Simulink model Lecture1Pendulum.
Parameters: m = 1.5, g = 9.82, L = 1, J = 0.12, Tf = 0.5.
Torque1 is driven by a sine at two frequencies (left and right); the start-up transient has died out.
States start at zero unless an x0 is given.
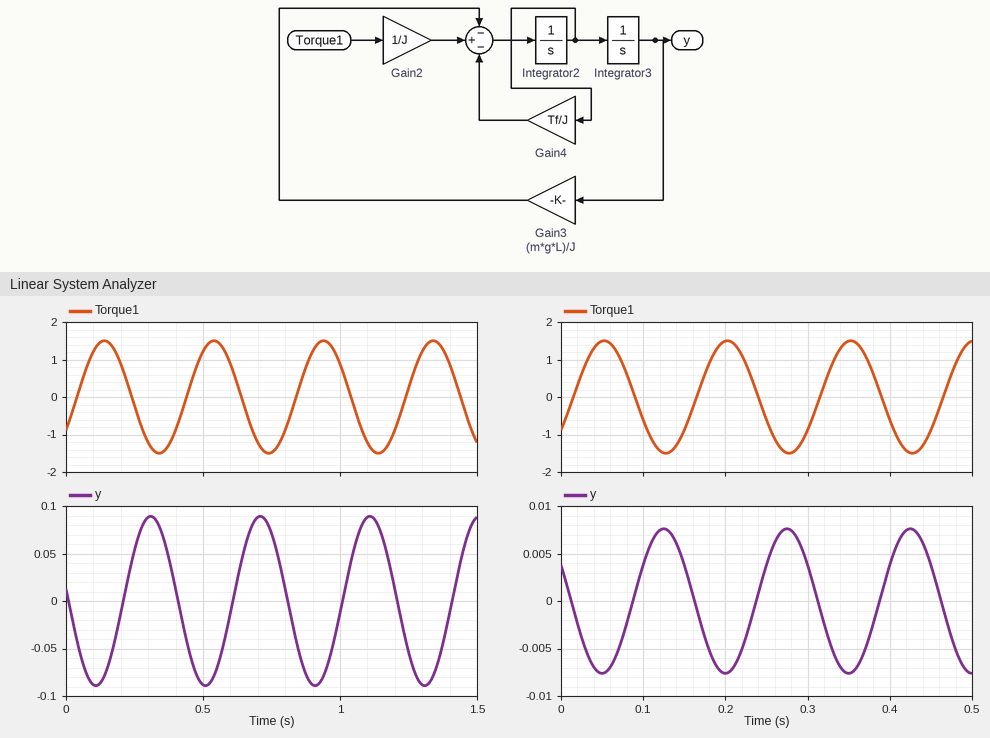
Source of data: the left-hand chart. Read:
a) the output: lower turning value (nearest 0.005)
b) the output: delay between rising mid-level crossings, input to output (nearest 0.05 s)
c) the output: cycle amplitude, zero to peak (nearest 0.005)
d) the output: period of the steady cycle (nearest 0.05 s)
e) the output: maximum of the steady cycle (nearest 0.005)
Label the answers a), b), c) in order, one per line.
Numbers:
a) -0.090
b) 0.15 s
c) 0.090
d) 0.40 s
e) 0.090
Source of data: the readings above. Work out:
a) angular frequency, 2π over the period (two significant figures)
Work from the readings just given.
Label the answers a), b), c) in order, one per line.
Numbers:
a) 16 rad/s
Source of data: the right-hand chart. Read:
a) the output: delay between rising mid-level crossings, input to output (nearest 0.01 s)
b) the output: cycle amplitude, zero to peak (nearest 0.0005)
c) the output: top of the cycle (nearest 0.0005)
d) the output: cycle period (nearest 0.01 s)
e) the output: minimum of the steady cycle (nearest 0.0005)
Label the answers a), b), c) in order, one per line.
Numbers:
a) 0.07 s
b) 0.0075
c) 0.0075
d) 0.15 s
e) -0.0075
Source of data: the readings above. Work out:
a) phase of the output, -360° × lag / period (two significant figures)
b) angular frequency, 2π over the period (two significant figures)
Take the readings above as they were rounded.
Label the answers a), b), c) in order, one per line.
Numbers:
a) -170°
b) 42 rad/s
